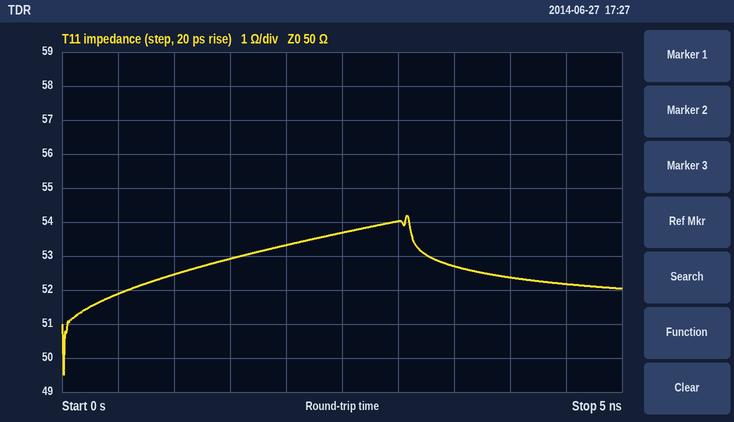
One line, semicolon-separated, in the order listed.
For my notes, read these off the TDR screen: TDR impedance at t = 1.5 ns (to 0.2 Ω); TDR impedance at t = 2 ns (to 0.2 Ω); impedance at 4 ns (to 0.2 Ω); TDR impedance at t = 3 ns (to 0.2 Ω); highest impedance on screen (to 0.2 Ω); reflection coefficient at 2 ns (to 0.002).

53.0 Ω; 53.4 Ω; 52.4 Ω; 54.0 Ω; 54.2 Ω; +0.032
